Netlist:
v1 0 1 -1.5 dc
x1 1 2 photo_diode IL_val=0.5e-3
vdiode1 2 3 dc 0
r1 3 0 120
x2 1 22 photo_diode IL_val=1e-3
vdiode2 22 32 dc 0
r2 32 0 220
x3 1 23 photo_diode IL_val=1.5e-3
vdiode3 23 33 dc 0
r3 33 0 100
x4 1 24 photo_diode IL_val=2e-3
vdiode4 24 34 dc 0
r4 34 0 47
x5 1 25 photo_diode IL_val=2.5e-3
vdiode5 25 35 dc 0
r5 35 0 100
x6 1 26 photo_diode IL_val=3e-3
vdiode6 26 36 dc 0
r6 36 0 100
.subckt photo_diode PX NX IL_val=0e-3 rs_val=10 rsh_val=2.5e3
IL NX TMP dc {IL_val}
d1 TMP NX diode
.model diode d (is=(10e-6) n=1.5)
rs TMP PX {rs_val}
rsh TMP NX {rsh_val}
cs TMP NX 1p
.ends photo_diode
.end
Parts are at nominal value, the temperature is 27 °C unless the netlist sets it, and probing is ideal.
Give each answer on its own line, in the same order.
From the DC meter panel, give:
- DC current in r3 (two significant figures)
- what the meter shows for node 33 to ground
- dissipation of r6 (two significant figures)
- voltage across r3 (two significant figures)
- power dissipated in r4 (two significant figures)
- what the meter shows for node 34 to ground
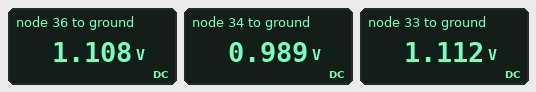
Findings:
11 mA
1.112 V
12 mW
1.1 V
21 mW
0.989 V
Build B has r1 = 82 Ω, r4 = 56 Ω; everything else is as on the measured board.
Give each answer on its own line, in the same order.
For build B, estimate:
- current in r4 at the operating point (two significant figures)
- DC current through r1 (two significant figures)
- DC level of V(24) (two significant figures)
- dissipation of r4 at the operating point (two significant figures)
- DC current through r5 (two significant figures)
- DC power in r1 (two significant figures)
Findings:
18 mA
13 mA
1.0 V
19 mW
11 mA
14 mW
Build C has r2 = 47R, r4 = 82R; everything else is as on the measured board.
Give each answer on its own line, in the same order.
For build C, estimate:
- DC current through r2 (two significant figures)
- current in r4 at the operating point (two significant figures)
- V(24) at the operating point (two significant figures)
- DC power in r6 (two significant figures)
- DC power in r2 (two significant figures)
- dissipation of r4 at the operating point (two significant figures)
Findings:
21 mA
13 mA
1.1 V
12 mW
21 mW
14 mW
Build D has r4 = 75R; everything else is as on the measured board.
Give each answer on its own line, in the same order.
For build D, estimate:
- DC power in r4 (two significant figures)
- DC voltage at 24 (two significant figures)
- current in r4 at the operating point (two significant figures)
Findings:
15 mW
1.1 V
14 mA
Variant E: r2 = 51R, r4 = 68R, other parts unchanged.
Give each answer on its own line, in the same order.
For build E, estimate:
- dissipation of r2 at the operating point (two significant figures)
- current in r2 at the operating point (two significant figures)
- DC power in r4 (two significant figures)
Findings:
20 mW
20 mA
16 mW
